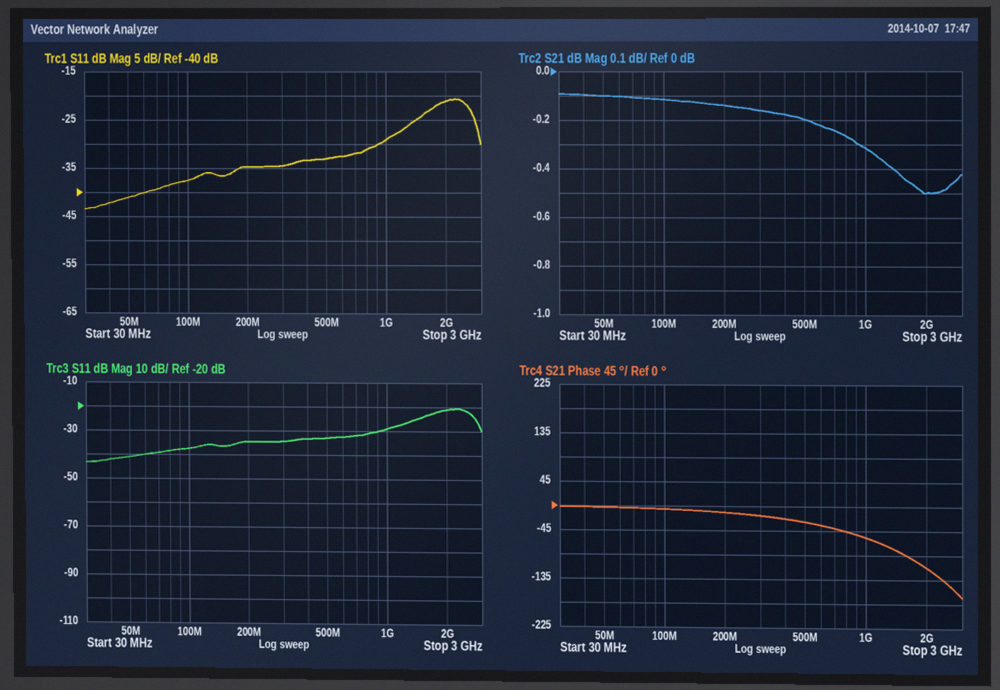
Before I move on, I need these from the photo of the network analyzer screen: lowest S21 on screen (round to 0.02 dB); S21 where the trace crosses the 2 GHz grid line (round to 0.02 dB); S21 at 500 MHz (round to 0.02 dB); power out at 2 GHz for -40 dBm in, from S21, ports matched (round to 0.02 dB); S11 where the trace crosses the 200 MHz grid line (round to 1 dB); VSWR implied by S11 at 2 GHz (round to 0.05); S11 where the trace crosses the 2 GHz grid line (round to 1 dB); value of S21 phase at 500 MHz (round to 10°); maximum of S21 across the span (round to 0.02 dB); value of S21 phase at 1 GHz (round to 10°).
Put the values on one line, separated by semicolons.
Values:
-0.50 dB; -0.50 dB; -0.20 dB; -40.50 dBm; -35 dB; 1.20; -21 dB; -30°; -0.10 dB; -60°
